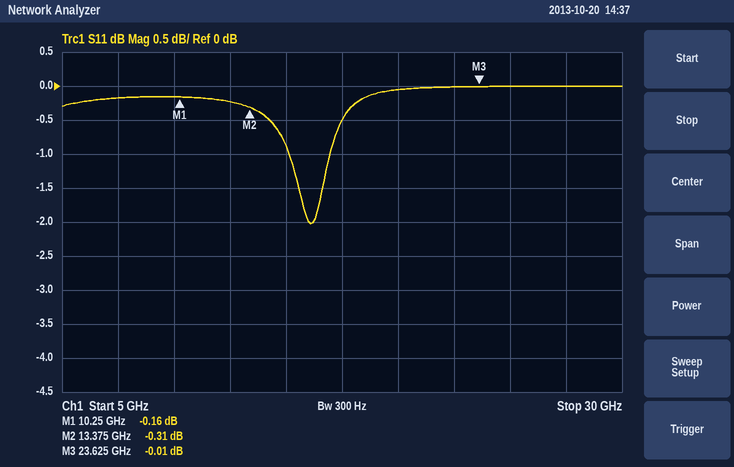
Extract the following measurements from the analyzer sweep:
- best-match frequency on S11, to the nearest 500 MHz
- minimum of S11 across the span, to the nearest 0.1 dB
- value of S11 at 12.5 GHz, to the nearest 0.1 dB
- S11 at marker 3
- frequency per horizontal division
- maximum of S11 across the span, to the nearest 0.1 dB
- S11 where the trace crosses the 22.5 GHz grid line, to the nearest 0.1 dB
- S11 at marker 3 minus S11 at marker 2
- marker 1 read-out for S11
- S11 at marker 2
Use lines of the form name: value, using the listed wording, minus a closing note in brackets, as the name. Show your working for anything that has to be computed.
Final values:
best-match frequency on S11, to the nearest 500 MHz: 16.0 GHz
minimum of S11 across the span, to the nearest 0.1 dB: -2.0 dB
value of S11 at 12.5 GHz, to the nearest 0.1 dB: -0.2 dB
S11 at marker 3: -0.01 dB
frequency per horizontal division: 2.5 GHz
maximum of S11 across the span, to the nearest 0.1 dB: 0.0 dB
S11 where the trace crosses the 22.5 GHz grid line, to the nearest 0.1 dB: 0.0 dB
S11 at marker 3 minus S11 at marker 2: -0.01 − (-0.31) = 0.30 dB
marker 1 read-out for S11: -0.16 dB
S11 at marker 2: -0.31 dB
